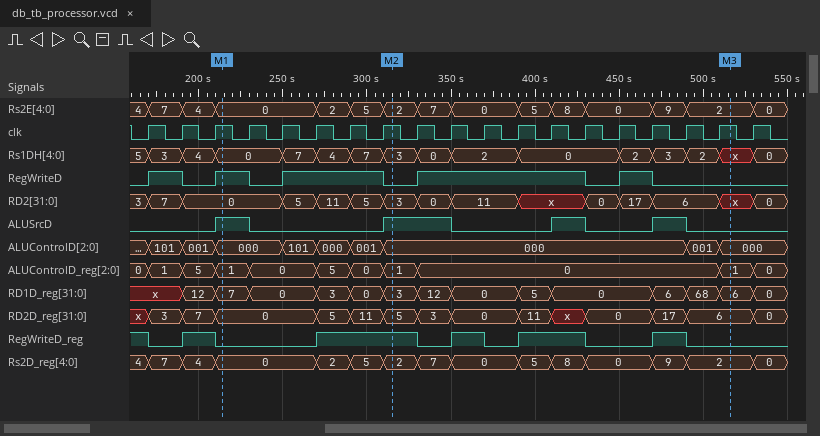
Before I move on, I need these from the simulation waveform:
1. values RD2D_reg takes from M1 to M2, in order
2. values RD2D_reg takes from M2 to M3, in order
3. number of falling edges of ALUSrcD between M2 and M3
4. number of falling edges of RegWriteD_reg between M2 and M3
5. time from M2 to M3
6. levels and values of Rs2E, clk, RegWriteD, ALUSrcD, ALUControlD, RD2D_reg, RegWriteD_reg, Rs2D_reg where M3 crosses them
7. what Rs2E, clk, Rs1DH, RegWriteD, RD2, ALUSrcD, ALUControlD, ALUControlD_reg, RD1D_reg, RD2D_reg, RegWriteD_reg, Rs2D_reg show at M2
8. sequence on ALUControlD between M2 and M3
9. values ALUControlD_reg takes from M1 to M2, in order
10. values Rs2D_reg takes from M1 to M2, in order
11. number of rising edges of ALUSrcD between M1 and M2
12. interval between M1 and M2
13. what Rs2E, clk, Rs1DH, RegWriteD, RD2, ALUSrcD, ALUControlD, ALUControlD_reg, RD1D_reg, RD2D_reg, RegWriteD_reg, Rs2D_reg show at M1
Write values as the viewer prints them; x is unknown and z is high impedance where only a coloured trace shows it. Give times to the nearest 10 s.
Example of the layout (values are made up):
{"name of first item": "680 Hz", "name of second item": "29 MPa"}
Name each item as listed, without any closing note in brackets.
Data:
{"values RD2D_reg takes from M1 to M2, in order": "0, 5, 11, 5", "values RD2D_reg takes from M2 to M3, in order": "5, 3, 0, 11, x, 0, 17, 6", "number of falling edges of ALUSrcD between M2 and M3": "3", "number of falling edges of RegWriteD_reg between M2 and M3": "4", "time from M2 to M3": "200 s", "levels and values of Rs2E, clk, RegWriteD, ALUSrcD, ALUControlD, RD2D_reg, RegWriteD_reg, Rs2D_reg where M3 crosses them": "Rs2E=2, clk=1, RegWriteD=0, ALUSrcD=0, ALUControlD=000, RD2D_reg=6, RegWriteD_reg=0, Rs2D_reg=2", "what Rs2E, clk, Rs1DH, RegWriteD, RD2, ALUSrcD, ALUControlD, ALUControlD_reg, RD1D_reg, RD2D_reg, RegWriteD_reg, Rs2D_reg show at M2": "Rs2E=2, clk=1, Rs1DH=3, RegWriteD=0, RD2=3, ALUSrcD=1, ALUControlD=000, ALUControlD_reg=1, RD1D_reg=3, RD2D_reg=5, RegWriteD_reg=1, Rs2D_reg=2", "sequence on ALUControlD between M2 and M3": "000, 001, 000", "values ALUControlD_reg takes from M1 to M2, in order": "1, 0, 5, 0, 1", "values Rs2D_reg takes from M1 to M2, in order": "0, 2, 5, 2", "number of rising edges of ALUSrcD between M1 and M2": "1", "interval between M1 and M2": "100 s", "what Rs2E, clk, Rs1DH, RegWriteD, RD2, ALUSrcD, ALUControlD, ALUControlD_reg, RD1D_reg, RD2D_reg, RegWriteD_reg, Rs2D_reg show at M1": "Rs2E=0, clk=1, Rs1DH=0, RegWriteD=1, RD2=0, ALUSrcD=1, ALUControlD=000, ALUControlD_reg=1, RD1D_reg=7, RD2D_reg=0, RegWriteD_reg=0, Rs2D_reg=0"}
